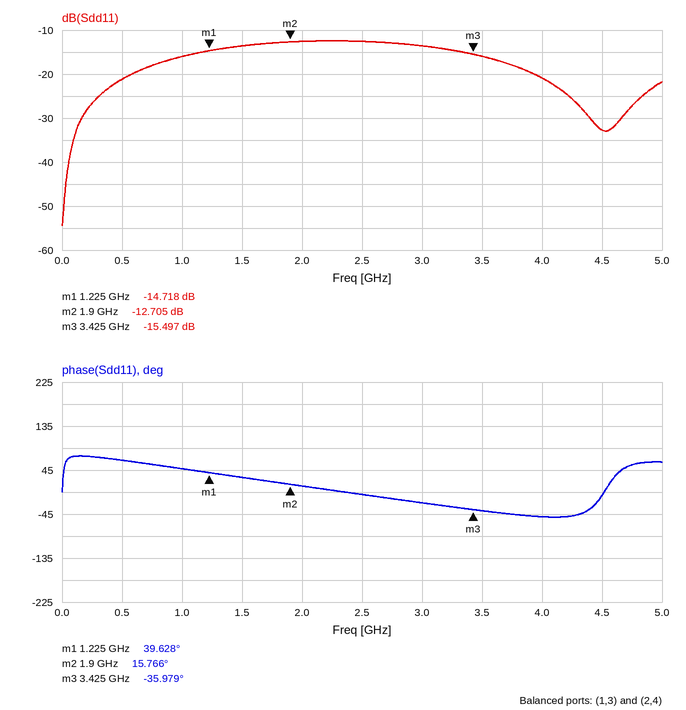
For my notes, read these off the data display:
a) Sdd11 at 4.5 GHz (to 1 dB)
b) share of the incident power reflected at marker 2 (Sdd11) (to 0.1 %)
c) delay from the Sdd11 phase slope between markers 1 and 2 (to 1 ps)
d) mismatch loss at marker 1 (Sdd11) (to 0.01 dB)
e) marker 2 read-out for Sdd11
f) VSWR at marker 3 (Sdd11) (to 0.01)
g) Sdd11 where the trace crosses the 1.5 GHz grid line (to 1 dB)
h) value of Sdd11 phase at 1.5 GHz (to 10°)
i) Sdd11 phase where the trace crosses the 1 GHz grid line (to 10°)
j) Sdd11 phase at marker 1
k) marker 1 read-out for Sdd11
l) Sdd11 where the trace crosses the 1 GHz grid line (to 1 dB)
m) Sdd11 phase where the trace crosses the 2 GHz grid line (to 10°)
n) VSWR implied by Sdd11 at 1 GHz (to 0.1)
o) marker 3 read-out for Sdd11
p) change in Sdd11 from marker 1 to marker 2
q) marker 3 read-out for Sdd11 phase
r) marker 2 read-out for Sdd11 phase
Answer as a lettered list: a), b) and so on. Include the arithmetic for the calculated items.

a) -33 dB
b) 10^(-12.705/10) ≈ 5.4 %
c) −(15.766° − (39.628°))/(360° × 675 MHz) ≈ 98 ps
d) −10 log10(1 − 10^(-14.718/10)) ≈ 0.15 dB
e) -12.705 dB
f) (1 + 0.1679)/(1 − 0.1679) ≈ 1.40
g) -14 dB
h) 30°
i) 50°
j) 39.628°
k) -14.718 dB
l) -16 dB
m) 10°
n) |Γ| = 10^(-16/20) = 0.1585; VSWR = (1 + 0.1585)/(1 − 0.1585) ≈ 1.4
o) -15.497 dB
p) -12.705 − (-14.718) = 2.013 dB
q) -35.979°
r) 15.766°
